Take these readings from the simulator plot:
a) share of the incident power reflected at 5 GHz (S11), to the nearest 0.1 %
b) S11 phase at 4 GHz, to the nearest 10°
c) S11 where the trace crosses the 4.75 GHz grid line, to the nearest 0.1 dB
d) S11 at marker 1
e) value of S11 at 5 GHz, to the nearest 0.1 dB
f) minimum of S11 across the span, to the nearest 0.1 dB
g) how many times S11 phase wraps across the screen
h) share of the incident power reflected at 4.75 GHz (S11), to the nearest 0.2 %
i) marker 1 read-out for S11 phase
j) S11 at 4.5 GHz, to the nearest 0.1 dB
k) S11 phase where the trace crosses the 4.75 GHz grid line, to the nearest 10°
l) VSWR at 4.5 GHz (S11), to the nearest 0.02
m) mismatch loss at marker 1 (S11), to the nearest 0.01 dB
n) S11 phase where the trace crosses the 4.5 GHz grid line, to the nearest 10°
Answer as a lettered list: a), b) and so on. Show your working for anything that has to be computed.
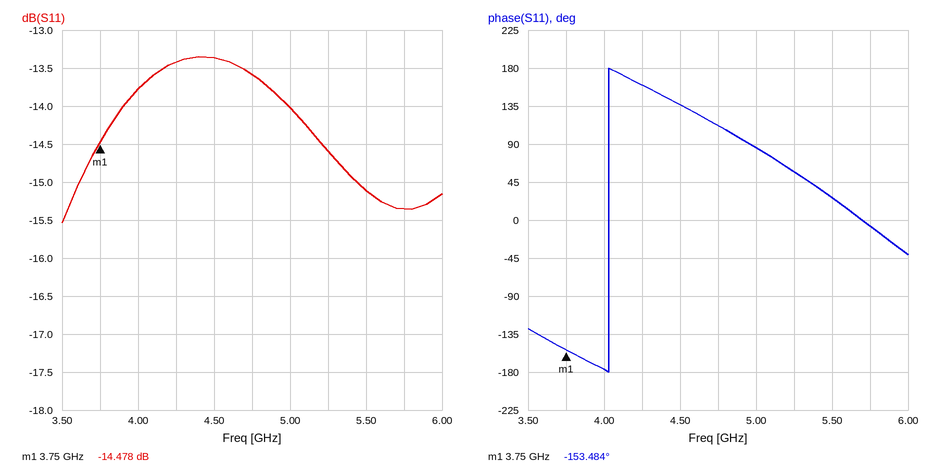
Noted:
a) 10^(-14/10) ≈ 4.0 %
b) -180°
c) -13.6 dB
d) -14.478 dB
e) -14.0 dB
f) -15.5 dB
g) 1
h) 10^(-13.6/10) ≈ 4.4 %
i) -153.484°
j) -13.4 dB
k) 110°
l) |Γ| = 10^(-13.4/20) = 0.2138; VSWR = (1 + 0.2138)/(1 − 0.2138) ≈ 1.54
m) −10 log10(1 − 10^(-14.478/10)) ≈ 0.16 dB
n) 140°
